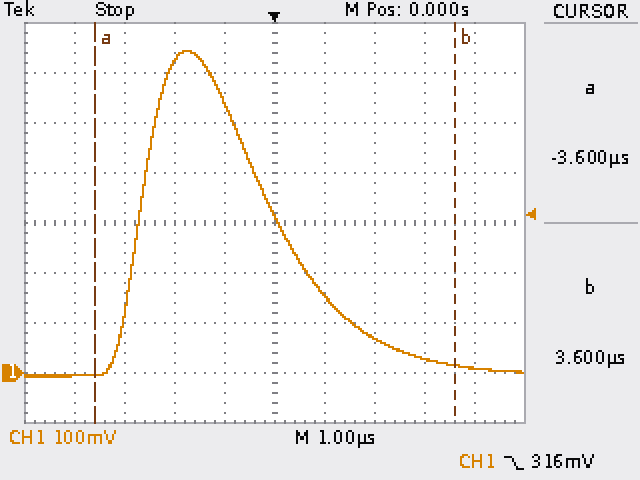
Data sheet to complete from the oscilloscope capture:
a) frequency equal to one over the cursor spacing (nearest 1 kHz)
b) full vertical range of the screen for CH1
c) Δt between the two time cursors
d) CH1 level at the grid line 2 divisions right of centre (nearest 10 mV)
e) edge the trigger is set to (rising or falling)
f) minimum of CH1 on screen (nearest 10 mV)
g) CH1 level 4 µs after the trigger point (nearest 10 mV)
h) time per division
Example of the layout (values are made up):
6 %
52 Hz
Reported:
139 kHz
800 mV
7.2 µs
70 mV
falling
-10 mV
10 mV
1 µs
